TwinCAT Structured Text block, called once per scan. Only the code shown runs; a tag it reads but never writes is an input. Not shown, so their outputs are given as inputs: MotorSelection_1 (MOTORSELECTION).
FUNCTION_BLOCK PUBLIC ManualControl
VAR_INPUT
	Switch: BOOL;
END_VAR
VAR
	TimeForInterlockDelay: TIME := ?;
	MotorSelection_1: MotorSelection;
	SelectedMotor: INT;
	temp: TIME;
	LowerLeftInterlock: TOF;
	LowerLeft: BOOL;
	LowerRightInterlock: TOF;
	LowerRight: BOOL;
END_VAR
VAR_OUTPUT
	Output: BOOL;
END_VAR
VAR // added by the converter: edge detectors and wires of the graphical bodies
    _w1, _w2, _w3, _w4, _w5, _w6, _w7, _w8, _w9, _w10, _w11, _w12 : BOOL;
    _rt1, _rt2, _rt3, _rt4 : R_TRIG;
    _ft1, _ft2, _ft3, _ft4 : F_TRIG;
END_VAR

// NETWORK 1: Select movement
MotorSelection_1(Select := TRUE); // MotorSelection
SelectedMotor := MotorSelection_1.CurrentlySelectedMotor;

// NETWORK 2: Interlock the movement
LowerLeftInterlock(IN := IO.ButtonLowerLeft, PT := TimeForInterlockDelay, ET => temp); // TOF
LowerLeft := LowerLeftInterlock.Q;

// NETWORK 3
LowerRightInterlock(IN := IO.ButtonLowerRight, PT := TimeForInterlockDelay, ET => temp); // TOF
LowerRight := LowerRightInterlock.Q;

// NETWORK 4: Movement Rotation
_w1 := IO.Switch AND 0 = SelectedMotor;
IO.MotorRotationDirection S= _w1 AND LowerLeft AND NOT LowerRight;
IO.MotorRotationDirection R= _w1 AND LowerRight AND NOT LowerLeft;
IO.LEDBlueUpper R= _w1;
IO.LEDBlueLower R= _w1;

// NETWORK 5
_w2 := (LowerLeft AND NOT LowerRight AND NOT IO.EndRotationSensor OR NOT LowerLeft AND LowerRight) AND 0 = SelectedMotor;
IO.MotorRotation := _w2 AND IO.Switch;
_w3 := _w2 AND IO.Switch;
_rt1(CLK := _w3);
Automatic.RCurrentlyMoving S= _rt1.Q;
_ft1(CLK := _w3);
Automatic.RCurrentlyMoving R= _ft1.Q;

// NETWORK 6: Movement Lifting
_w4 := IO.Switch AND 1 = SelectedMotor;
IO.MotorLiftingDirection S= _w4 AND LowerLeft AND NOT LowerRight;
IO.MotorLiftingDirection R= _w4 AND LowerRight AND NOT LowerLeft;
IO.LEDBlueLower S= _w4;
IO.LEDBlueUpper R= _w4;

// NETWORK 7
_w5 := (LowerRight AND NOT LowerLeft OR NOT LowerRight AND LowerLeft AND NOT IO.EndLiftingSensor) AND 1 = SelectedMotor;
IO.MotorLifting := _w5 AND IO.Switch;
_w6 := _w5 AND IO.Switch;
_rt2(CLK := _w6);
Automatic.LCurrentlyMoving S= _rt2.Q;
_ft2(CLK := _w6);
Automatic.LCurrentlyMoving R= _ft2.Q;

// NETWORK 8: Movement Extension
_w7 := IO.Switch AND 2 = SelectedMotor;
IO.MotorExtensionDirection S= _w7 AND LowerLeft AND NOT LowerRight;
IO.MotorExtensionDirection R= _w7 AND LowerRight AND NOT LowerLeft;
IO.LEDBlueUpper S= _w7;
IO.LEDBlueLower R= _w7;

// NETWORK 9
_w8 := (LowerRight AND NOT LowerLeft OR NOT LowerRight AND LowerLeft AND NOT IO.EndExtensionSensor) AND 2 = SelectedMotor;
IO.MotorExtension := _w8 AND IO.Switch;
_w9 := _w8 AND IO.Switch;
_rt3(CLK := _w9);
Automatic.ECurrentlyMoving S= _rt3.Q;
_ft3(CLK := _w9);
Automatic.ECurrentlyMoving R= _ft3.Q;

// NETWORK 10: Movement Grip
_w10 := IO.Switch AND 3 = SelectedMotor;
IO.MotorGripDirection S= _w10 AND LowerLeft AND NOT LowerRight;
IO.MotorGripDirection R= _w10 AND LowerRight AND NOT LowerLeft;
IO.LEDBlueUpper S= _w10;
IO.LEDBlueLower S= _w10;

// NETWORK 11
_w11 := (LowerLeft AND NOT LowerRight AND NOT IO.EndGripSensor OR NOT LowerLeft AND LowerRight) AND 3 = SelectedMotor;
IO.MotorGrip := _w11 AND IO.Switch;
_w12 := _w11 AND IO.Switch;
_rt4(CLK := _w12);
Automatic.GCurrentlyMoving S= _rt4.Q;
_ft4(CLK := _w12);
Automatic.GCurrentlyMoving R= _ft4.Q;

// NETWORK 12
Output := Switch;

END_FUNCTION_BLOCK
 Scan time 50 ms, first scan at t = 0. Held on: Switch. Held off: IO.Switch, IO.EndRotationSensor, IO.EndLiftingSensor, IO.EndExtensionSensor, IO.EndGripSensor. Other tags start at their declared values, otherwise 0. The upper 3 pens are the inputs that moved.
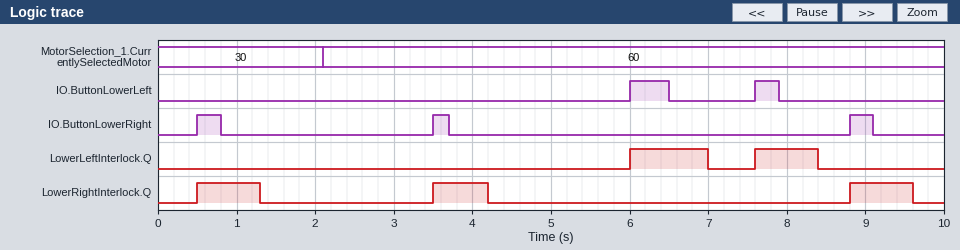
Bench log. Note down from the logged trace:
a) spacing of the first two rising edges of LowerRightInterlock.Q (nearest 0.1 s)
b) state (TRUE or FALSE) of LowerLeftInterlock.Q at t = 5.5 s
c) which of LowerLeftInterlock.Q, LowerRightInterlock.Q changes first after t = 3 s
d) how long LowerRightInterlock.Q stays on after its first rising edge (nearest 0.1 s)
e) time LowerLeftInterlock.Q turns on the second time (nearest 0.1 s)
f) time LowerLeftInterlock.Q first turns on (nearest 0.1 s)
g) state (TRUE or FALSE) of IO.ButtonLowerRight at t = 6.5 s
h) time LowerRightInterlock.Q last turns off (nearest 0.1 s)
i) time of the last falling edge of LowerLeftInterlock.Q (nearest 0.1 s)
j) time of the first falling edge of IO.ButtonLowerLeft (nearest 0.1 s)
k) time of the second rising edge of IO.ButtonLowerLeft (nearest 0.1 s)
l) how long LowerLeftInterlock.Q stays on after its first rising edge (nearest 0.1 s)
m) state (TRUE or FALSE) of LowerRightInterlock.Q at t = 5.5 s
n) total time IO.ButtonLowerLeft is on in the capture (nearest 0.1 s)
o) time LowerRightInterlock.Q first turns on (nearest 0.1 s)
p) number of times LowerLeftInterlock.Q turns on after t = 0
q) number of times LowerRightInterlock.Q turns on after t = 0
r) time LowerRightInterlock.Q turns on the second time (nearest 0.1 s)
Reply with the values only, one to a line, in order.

3.0 s
FALSE
LowerRightInterlock.Q
0.8 s
7.6 s
6.0 s
FALSE
9.6 s
8.4 s
6.5 s
7.6 s
1.0 s
FALSE
0.8 s
0.5 s
2
3
3.5 s
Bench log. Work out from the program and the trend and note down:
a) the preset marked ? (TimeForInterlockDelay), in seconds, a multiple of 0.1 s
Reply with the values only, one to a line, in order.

0.5 s
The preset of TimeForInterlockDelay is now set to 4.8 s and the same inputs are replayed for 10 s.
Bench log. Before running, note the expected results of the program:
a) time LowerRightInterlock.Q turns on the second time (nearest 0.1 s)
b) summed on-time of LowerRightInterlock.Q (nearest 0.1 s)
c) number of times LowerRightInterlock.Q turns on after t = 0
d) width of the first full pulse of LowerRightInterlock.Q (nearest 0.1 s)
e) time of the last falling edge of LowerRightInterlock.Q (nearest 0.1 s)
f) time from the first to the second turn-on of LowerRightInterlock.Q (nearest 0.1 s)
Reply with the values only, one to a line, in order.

8.8 s
9.2 s
2
8.0 s
8.5 s
8.3 s
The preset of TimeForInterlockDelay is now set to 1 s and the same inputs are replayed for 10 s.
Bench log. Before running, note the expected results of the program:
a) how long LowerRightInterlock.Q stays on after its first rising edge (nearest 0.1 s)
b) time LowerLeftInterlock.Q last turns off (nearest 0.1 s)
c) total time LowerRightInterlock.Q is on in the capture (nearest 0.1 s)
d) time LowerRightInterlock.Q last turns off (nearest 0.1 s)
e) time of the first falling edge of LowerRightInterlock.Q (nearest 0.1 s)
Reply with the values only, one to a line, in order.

1.3 s
8.9 s
3.7 s
4.7 s
1.8 s
